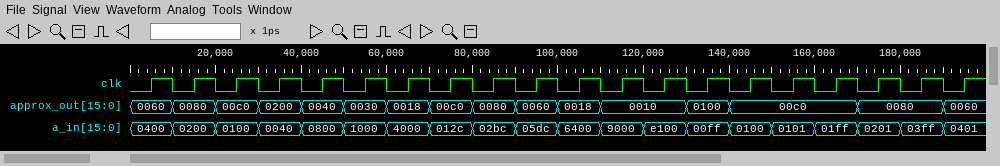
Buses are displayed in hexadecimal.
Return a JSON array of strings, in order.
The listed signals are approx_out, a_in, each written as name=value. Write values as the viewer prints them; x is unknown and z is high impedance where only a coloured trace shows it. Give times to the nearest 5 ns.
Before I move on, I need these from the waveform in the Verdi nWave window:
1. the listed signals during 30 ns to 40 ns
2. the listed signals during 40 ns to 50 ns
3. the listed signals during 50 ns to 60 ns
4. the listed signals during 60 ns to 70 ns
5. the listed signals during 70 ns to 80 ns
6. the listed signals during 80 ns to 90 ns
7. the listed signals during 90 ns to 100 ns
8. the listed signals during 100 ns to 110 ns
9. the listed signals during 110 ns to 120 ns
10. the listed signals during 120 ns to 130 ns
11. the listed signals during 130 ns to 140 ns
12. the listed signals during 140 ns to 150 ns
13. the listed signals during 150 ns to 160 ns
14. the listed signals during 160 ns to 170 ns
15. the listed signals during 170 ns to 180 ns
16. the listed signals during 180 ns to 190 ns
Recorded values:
["approx_out=0200, a_in=0040", "approx_out=0040, a_in=0800", "approx_out=0030, a_in=1000", "approx_out=0018, a_in=4000", "approx_out=00c0, a_in=012c", "approx_out=0080, a_in=02bc", "approx_out=0060, a_in=05dc", "approx_out=0018, a_in=6400", "approx_out=0010, a_in=9000", "approx_out=0010, a_in=e100", "approx_out=0100, a_in=00ff", "approx_out=00c0, a_in=0100", "approx_out=00c0, a_in=0101", "approx_out=00c0, a_in=01ff", "approx_out=0080, a_in=0201", "approx_out=0080, a_in=03ff"]
